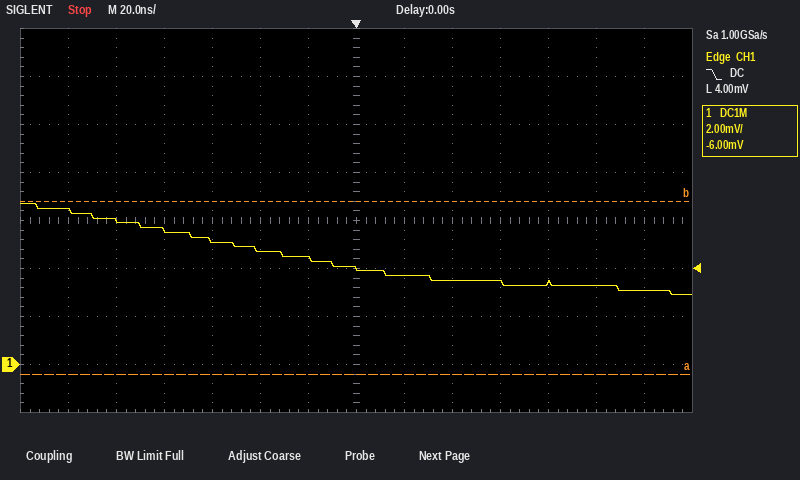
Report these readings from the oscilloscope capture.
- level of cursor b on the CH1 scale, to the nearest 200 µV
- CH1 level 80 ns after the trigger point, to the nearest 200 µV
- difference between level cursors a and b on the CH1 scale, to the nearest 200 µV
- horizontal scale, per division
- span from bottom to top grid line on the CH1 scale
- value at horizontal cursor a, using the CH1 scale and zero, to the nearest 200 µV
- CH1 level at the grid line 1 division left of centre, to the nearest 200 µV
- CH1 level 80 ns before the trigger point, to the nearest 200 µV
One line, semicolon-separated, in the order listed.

6.8 mV; 3.4 mV; 7.2 mV; 20 ns; 16 mV; -400 µV; 4.4 mV; 5.6 mV
